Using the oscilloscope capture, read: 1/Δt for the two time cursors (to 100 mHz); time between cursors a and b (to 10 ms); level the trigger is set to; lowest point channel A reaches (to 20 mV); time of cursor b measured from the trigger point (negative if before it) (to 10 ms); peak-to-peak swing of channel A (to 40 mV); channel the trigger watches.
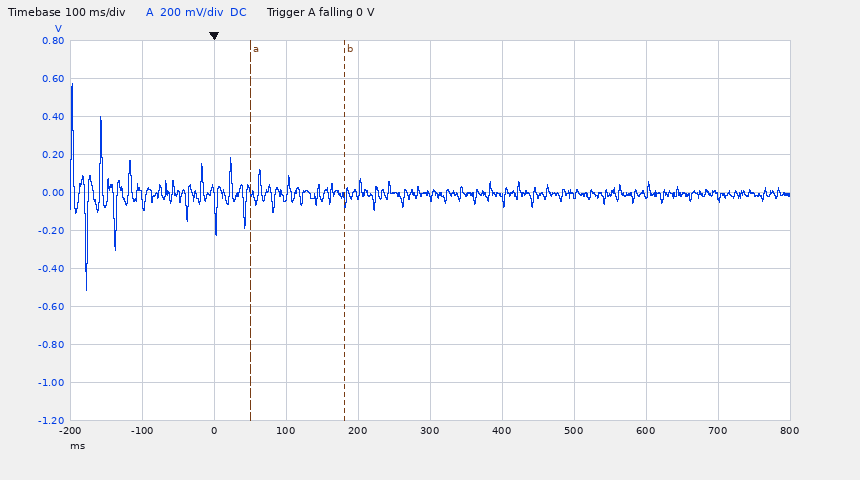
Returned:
7.7 Hz
130 ms
0 V
-520 mV
+180 ms
1.08 V
channel A
